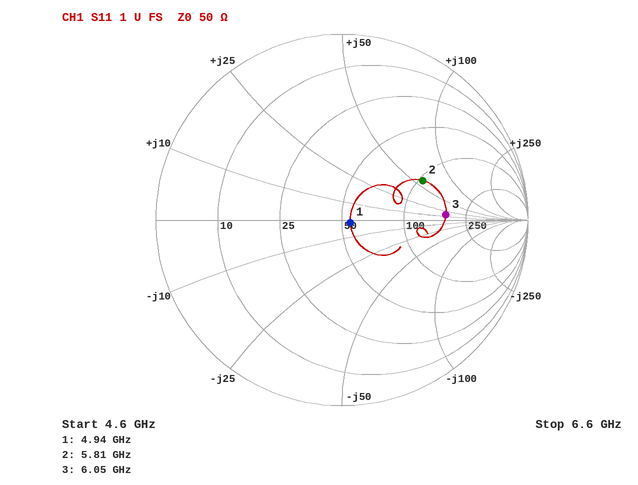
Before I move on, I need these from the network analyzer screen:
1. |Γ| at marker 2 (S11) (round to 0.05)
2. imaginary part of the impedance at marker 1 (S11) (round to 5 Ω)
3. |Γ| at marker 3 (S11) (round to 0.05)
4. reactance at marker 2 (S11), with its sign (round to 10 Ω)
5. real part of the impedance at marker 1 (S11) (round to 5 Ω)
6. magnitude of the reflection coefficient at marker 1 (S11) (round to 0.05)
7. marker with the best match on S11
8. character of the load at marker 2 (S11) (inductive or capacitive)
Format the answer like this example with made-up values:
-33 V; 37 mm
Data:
0.50; 0 Ω; 0.55; +60 Ω; 55 Ω; 0.05; marker 1; inductive
